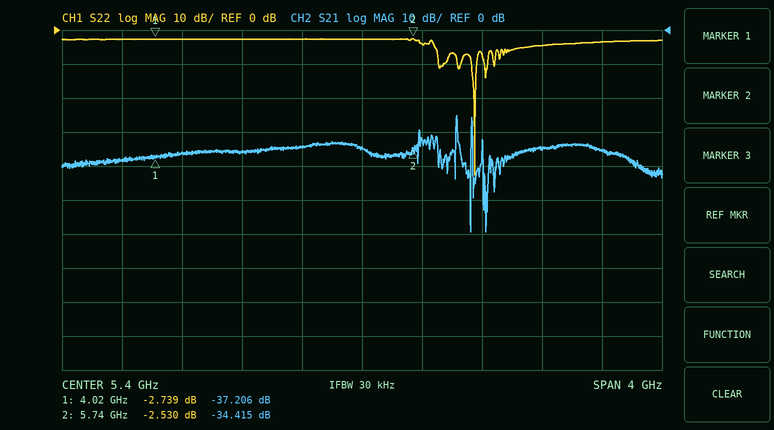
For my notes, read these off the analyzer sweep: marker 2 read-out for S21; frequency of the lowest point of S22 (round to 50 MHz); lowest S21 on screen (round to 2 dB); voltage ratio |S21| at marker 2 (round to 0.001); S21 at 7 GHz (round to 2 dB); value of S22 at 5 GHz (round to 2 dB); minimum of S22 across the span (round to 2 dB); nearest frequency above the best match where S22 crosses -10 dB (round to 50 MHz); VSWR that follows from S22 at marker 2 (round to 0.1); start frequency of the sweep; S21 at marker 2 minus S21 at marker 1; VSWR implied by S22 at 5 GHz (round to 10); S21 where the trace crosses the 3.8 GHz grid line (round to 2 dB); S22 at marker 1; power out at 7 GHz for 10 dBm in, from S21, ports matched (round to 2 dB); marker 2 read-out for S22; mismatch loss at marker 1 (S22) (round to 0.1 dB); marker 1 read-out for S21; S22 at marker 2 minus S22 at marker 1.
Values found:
-34.415 dB
6.15 GHz
-60 dB
0.019
-36 dB
-2 dB
-42 dB
6.15 GHz
6.9
3.4 GHz
2.791 dB
10
-38 dB
-2.739 dB
-26 dBm
-2.530 dB
3.3 dB
-37.206 dB
0.209 dB
